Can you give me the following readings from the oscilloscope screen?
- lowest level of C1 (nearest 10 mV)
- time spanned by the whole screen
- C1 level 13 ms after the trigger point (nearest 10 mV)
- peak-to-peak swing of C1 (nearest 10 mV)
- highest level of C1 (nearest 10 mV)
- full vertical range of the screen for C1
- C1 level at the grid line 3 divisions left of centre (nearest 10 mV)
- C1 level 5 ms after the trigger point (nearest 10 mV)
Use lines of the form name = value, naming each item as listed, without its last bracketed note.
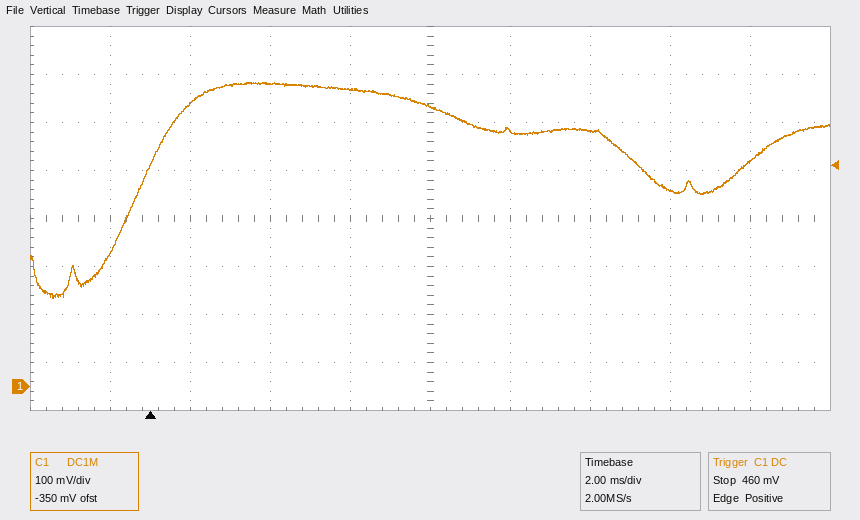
lowest level of C1 = 180 mV
time spanned by the whole screen = 20 ms
C1 level 13 ms after the trigger point = 410 mV
peak-to-peak swing of C1 = 450 mV
highest level of C1 = 630 mV
full vertical range of the screen for C1 = 800 mV
C1 level at the grid line 3 divisions left of centre = 590 mV
C1 level 5 ms after the trigger point = 620 mV
